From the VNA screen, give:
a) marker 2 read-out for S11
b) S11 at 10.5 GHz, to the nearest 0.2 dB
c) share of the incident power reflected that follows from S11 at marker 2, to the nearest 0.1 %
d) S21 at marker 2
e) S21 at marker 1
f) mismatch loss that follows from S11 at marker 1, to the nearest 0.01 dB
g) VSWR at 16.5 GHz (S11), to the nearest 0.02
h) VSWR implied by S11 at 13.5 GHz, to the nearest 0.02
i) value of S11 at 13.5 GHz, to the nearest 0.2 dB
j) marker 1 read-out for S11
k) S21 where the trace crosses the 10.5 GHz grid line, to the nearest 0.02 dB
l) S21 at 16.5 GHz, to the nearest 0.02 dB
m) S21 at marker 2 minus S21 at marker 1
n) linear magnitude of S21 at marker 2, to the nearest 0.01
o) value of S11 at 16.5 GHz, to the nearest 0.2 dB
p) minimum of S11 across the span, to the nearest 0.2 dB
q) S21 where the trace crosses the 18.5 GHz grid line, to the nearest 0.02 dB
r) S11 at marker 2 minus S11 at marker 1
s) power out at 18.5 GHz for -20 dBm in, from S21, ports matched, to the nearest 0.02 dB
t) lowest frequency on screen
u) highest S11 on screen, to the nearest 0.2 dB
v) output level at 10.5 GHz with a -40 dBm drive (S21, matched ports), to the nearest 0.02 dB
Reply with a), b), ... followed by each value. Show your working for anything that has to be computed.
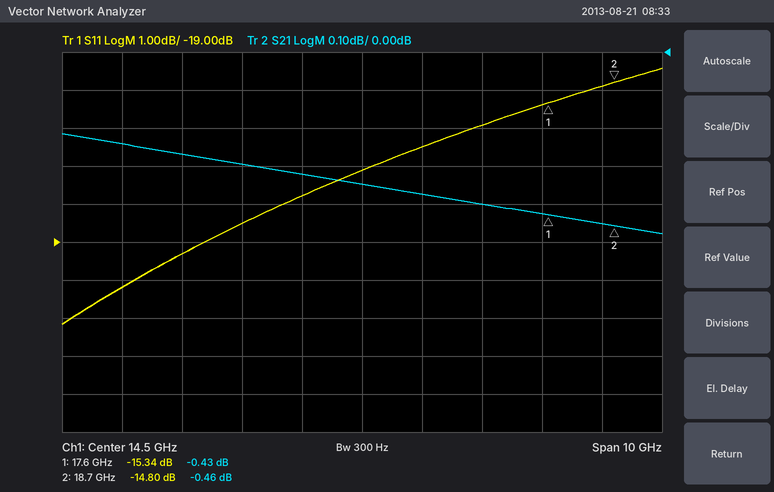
a) -14.80 dB
b) -20.2 dB
c) 10^(-14.8/10) ≈ 3.3 %
d) -0.46 dB
e) -0.43 dB
f) −10 log10(1 − 10^(-15.34/10)) ≈ 0.13 dB
g) |Γ| = 10^(-16/20) = 0.1585; VSWR = (1 + 0.1585)/(1 − 0.1585) ≈ 1.38
h) |Γ| = 10^(-17.8/20) = 0.1288; VSWR = (1 + 0.1288)/(1 − 0.1288) ≈ 1.30
i) -17.8 dB
j) -15.34 dB
k) -0.24 dB
l) -0.40 dB
m) -0.46 − (-0.43) = -0.03 dB
n) 10^(-0.46/20) ≈ 0.95
o) -16.0 dB
p) -21.2 dB
q) -0.46 dB
r) -14.8 − (-15.34) = 0.54 dB
s) -20 dBm + (-0.46 dB) = -20.46 dBm
t) 9.5 GHz
u) -14.4 dB
v) -40 dBm + (-0.24 dB) = -40.24 dBm
